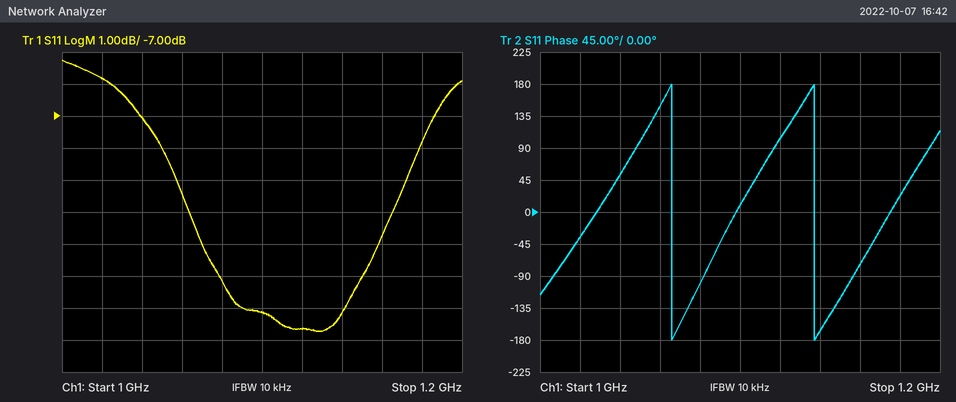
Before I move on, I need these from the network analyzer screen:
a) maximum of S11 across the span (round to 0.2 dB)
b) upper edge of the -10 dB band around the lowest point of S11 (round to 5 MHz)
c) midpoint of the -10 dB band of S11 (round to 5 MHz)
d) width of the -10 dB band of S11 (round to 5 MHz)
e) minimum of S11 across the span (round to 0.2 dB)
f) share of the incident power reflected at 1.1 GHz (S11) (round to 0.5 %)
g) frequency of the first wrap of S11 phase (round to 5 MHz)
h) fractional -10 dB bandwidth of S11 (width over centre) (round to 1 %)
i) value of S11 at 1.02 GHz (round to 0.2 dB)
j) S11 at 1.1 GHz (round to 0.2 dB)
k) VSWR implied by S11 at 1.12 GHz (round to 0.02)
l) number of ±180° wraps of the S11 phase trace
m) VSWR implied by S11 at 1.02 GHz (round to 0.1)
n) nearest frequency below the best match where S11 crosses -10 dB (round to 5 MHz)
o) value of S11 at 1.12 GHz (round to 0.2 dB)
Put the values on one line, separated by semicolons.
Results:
-5.2 dB; 1.165 GHz; 1.115 GHz; 100 MHz; -13.8 dB; 5.0 %; 1.065 GHz; 9 %; -5.8 dB; -13.2 dB; 1.52; 2; 3.1; 1.065 GHz; -13.6 dB
